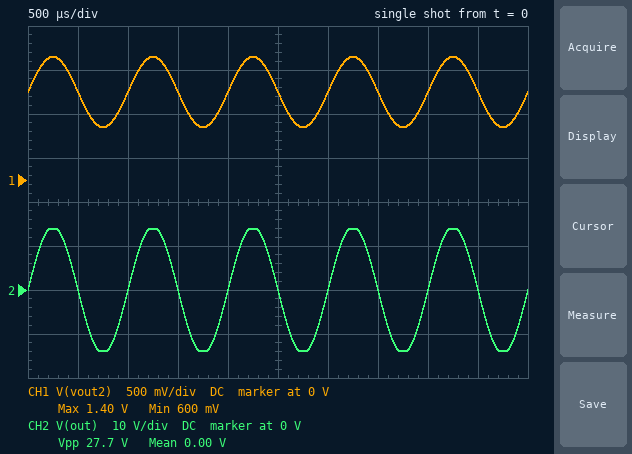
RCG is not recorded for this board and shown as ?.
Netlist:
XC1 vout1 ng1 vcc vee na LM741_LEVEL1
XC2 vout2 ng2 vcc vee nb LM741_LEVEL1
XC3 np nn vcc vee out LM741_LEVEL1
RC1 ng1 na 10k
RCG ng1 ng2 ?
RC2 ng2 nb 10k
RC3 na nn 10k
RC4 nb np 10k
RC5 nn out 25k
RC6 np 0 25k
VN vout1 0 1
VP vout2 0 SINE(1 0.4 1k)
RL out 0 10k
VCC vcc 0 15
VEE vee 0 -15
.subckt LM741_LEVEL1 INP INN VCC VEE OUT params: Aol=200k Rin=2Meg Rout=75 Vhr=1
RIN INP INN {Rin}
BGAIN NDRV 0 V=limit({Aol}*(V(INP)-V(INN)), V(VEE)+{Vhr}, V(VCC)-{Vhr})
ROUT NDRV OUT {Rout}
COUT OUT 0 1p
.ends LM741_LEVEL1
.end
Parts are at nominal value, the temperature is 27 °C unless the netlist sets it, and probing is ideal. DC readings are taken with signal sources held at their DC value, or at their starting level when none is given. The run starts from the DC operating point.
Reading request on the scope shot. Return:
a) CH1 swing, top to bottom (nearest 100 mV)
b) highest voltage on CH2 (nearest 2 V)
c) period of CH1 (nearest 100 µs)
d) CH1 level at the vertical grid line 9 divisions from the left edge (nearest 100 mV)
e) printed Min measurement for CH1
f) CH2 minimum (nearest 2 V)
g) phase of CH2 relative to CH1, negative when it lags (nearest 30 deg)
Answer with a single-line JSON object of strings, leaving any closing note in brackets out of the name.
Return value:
{"CH1 swing, top to bottom": "800 mV", "highest voltage on CH2": "14 V", "period of CH1": "1.0 ms", "CH1 level at the vertical grid line 9 divisions from the left edge": "1.0 V", "printed Min measurement for CH1": "600 mV", "CH2 minimum": "-14 V", "phase of CH2 relative to CH1, negative when it lags": "0 deg"}
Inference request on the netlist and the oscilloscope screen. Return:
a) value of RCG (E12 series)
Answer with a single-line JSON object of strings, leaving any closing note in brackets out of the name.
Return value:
{"value of RCG": "1.5 kΩ"}
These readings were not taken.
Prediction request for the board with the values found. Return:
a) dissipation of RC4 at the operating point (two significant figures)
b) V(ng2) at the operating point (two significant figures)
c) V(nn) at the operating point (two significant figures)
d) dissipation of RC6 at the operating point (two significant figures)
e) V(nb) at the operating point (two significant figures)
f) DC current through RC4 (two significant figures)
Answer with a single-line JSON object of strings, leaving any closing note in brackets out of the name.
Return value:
{"dissipation of RC4 at the operating point": "8.2 µW", "V(ng2) at the operating point": "1.0 V", "V(nn) at the operating point": "710 mV", "dissipation of RC6 at the operating point": "20 µW", "V(nb) at the operating point": "1.0 V", "DC current through RC4": "29 µA"}
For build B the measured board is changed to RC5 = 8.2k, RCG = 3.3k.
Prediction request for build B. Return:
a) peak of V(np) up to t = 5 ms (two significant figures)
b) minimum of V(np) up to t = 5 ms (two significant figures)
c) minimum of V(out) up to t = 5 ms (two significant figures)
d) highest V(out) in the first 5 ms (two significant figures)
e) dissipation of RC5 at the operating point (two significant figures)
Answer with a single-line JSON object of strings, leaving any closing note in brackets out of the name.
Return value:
{"peak of V(np) up to t = 5 ms": "1.9 V", "minimum of V(np) up to t = 5 ms": "-440 mV", "minimum of V(out) up to t = 5 ms": "-2.6 V", "highest V(out) in the first 5 ms": "3.6 V", "dissipation of RC5 at the operating point": "6.7 µW"}
